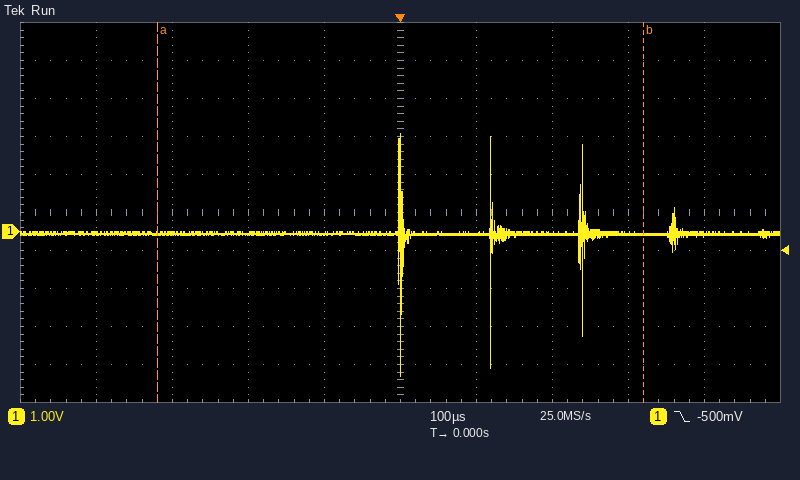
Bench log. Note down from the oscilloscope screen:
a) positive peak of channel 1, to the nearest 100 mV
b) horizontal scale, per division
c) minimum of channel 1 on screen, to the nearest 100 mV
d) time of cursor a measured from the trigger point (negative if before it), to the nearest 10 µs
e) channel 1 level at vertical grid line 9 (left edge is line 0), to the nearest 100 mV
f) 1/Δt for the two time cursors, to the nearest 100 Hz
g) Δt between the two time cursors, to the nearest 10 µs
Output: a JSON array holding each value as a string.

["2.6 V", "100 µs", "-3.8 V", "-320 µs", "-100 mV", "1.6 kHz", "640 µs"]
